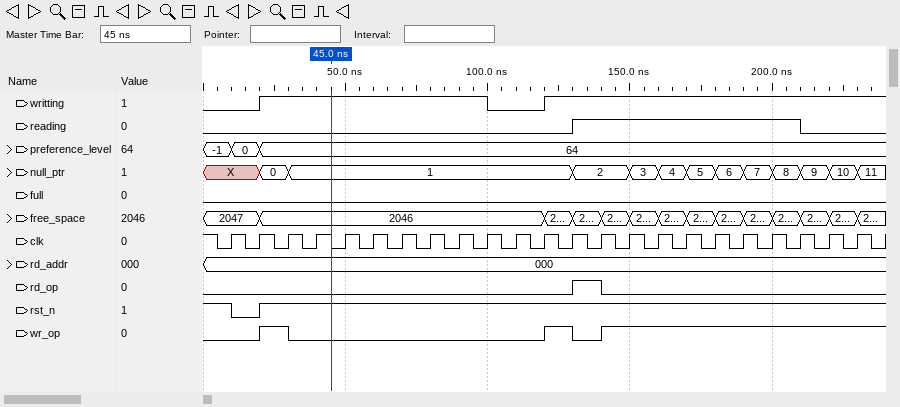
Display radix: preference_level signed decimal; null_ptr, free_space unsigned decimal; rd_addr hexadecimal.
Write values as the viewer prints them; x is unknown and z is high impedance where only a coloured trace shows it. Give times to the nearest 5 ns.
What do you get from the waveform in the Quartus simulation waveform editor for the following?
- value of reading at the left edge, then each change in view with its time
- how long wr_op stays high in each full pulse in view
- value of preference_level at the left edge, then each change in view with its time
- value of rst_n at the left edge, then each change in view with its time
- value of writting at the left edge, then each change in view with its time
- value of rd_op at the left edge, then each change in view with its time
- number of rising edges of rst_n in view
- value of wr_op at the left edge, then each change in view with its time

0, 1 at 130 ns, 0 at 210 ns
10 ns, 10 ns
-1, 0 at 10 ns, 64 at 20 ns
1, 0 at 10 ns, 1 at 20 ns
0, 1 at 20 ns, 0 at 100 ns, 1 at 120 ns
0, 1 at 130 ns, 0 at 140 ns
1
0, 1 at 20 ns, 0 at 30 ns, 1 at 120 ns, 0 at 130 ns, 1 at 140 ns
